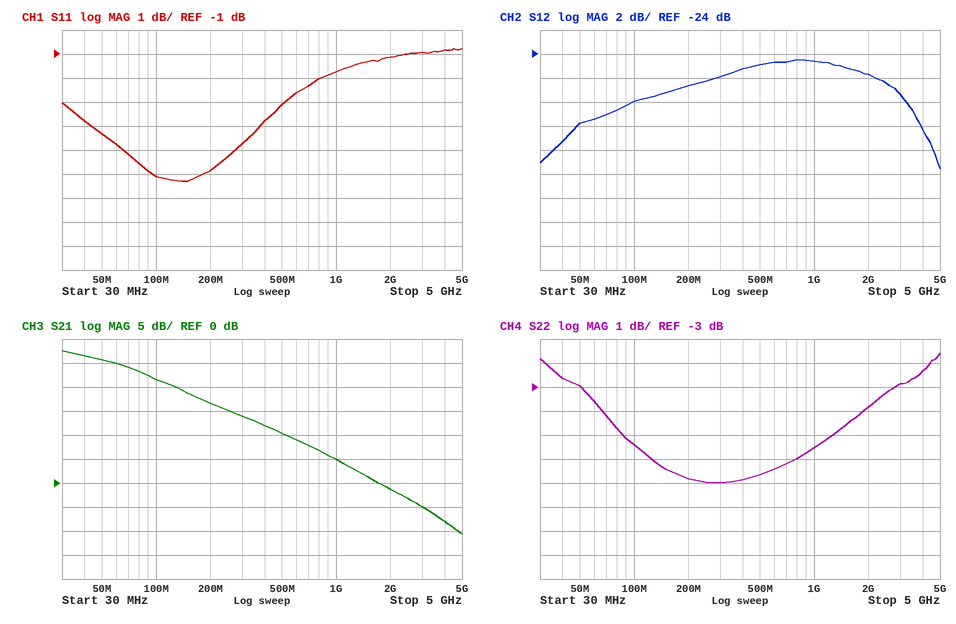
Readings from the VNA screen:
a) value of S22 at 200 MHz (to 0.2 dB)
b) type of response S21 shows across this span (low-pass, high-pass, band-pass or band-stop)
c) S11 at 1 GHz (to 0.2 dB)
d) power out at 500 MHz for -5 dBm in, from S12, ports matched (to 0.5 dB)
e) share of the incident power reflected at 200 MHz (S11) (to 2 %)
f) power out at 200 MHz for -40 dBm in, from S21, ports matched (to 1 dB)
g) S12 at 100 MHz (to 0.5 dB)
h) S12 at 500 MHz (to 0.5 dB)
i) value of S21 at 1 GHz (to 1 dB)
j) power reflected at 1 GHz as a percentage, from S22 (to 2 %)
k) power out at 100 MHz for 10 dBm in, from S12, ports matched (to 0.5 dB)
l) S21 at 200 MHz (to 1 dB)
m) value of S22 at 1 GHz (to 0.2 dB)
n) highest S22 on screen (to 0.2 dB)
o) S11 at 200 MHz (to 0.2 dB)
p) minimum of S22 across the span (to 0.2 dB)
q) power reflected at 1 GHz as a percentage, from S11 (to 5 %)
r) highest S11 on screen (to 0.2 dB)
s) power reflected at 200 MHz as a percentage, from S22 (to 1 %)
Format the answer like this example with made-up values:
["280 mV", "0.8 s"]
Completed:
["-6.8 dB", "low-pass", "-1.8 dB", "-30.0 dBm", "26 %", "-23 dBm", "-28.0 dB", "-25.0 dB", "5 dB", "28 %", "-18.0 dBm", "17 dB", "-5.6 dB", "-1.6 dB", "-5.8 dB", "-7.0 dB", "65 %", "-0.8 dB", "21 %"]
